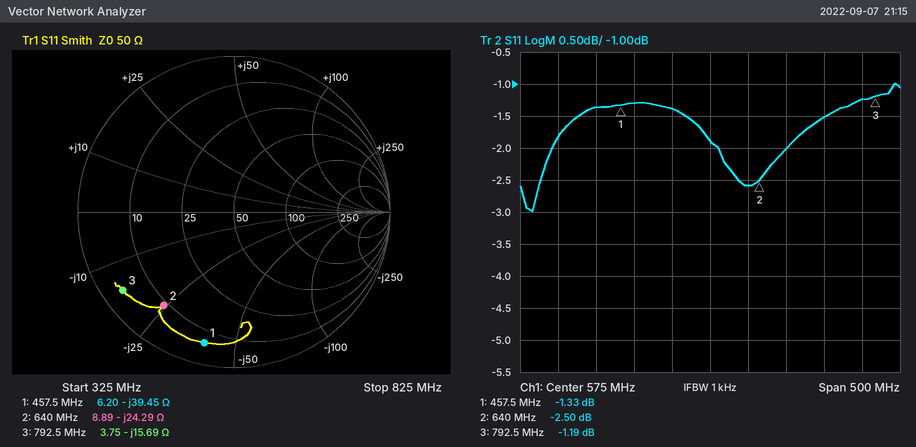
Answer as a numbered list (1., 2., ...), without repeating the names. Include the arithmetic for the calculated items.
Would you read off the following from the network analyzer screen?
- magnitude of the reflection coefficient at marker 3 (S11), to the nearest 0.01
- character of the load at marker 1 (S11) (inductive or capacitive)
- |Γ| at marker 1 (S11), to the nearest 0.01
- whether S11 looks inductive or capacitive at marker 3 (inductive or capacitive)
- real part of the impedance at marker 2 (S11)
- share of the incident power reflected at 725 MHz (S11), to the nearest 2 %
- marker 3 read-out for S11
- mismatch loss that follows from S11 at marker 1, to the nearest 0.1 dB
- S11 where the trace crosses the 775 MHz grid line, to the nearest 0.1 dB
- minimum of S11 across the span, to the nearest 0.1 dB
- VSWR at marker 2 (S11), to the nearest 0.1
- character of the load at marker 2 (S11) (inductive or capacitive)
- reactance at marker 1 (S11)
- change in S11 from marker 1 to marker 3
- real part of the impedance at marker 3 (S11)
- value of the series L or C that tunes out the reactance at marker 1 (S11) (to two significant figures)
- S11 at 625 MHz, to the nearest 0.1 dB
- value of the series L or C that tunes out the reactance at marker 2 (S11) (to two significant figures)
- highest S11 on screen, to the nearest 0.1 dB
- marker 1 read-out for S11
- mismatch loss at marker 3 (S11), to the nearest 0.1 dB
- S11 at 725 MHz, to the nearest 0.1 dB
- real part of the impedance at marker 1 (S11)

1. 0.87
2. capacitive
3. 0.86
4. capacitive
5. 8.89 Ω
6. 10^(-1.5/10) ≈ 70.8 %, so 70 % to the nearest 2 %
7. -1.19 dB
8. −10 log10(1 − 10^(-1.33/10)) ≈ 5.8 dB
9. -1.2 dB
10. -3.0 dB
11. 7.0
12. capacitive
13. -39.45 Ω
14. -1.19 − (-1.33) = 0.14 dB
15. 3.75 Ω
16. L = 39.45 Ω/(2π × 457.5 MHz) ≈ 14 nH
17. -2.6 dB
18. L = 24.29 Ω/(2π × 640 MHz) ≈ 6.0 nH
19. -1.0 dB
20. -1.33 dB
21. −10 log10(1 − 10^(-1.19/10)) ≈ 6.2 dB
22. -1.5 dB
23. 6.20 Ω
